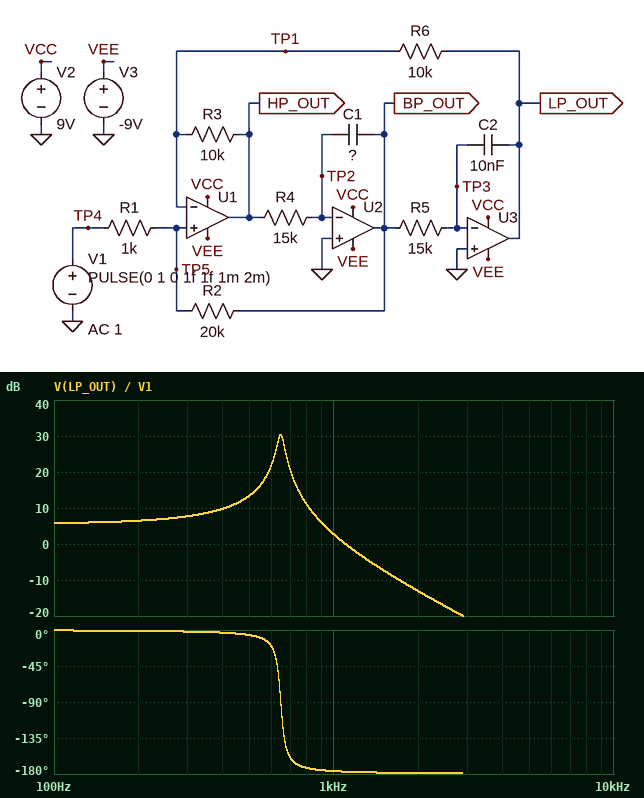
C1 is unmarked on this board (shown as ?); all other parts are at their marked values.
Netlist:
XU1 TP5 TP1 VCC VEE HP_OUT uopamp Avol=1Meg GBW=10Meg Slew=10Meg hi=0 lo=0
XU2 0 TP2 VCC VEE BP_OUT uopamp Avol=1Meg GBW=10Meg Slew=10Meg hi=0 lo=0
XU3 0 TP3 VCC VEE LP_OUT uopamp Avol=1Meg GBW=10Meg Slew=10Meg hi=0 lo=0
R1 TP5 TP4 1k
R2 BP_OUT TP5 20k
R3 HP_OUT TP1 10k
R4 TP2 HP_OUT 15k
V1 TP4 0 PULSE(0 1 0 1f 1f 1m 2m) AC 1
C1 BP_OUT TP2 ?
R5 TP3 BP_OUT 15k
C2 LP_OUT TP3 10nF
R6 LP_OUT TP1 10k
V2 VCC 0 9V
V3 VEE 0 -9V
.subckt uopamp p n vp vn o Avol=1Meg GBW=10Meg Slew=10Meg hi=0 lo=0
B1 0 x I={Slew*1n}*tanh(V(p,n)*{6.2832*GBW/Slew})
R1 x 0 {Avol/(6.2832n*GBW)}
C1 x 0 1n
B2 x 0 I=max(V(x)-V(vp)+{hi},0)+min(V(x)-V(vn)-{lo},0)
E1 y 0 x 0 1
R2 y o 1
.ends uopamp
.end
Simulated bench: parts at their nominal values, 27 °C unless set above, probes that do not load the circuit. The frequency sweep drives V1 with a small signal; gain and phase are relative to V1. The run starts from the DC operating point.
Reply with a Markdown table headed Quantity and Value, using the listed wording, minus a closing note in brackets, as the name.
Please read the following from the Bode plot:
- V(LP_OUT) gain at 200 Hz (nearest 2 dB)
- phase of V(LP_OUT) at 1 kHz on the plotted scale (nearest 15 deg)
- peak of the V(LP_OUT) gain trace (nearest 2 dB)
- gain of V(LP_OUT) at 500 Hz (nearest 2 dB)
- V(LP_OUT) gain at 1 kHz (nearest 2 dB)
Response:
| Quantity | Value |
|---|---|
| V(LP_OUT) gain at 200 Hz | 6 dB |
| phase of V(LP_OUT) at 1 kHz on the plotted scale | -180 deg |
| peak of the V(LP_OUT) gain trace | 30 dB |
| gain of V(LP_OUT) at 500 Hz | 14 dB |
| V(LP_OUT) gain at 1 kHz | 2 dB |
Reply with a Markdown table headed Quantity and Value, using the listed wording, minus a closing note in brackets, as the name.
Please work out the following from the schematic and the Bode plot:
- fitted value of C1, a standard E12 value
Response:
| Quantity | Value |
|---|---|
| fitted value of C1, a standard E12 value | 27 nF |
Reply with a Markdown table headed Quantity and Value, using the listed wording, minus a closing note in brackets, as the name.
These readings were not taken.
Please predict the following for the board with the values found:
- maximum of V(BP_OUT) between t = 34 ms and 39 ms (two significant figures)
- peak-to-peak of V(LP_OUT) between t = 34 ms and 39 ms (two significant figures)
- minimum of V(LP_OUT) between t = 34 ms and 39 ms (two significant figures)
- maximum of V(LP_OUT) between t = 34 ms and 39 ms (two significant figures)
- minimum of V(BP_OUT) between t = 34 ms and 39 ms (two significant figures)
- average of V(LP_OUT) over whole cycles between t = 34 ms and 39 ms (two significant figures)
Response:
| Quantity | Value |
|---|---|
| maximum of V(BP_OUT) between t = 34 ms and 39 ms | 1.4 V |
| peak-to-peak of V(LP_OUT) between t = 34 ms and 39 ms | 6.2 V |
| minimum of V(LP_OUT) between t = 34 ms and 39 ms | -2.2 V |
| maximum of V(LP_OUT) between t = 34 ms and 39 ms | 4.1 V |
| minimum of V(BP_OUT) between t = 34 ms and 39 ms | -1.4 V |
| average of V(LP_OUT) over whole cycles between t = 34 ms and 39 ms | 950 mV |
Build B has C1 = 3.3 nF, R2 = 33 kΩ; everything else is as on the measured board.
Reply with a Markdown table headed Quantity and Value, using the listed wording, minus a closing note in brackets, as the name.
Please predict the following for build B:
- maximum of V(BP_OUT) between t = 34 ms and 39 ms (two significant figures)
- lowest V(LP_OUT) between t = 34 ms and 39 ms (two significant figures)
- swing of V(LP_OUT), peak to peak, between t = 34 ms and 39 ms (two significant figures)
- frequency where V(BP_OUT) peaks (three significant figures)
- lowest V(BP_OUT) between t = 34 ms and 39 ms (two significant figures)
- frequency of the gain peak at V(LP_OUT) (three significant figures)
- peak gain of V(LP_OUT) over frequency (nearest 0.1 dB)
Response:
| Quantity | Value |
|---|---|
| maximum of V(BP_OUT) between t = 34 ms and 39 ms | 2.3 V |
| lowest V(LP_OUT) between t = 34 ms and 39 ms | -1.2 V |
| swing of V(LP_OUT), peak to peak, between t = 34 ms and 39 ms | 4.4 V |
| frequency where V(BP_OUT) peaks | 1.85 kHz |
| lowest V(BP_OUT) between t = 34 ms and 39 ms | -2.3 V |
| frequency of the gain peak at V(LP_OUT) | 1.84 kHz |
| peak gain of V(LP_OUT) over frequency | 25.6 dB |
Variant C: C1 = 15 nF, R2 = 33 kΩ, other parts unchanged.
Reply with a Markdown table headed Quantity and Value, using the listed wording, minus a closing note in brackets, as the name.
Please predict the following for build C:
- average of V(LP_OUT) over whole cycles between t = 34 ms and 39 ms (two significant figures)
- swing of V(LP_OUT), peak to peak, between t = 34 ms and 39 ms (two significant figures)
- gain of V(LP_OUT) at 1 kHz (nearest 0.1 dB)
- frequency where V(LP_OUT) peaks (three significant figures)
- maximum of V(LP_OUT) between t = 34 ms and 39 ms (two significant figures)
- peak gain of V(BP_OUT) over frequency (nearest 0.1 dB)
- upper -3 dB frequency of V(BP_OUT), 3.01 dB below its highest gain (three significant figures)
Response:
| Quantity | Value |
|---|---|
| average of V(LP_OUT) over whole cycles between t = 34 ms and 39 ms | 970 mV |
| swing of V(LP_OUT), peak to peak, between t = 34 ms and 39 ms | 4.1 V |
| gain of V(LP_OUT) at 1 kHz | 15.2 dB |
| frequency where V(LP_OUT) peaks | 866 Hz |
| maximum of V(LP_OUT) between t = 34 ms and 39 ms | 3.0 V |
| peak gain of V(BP_OUT) over frequency | 30.4 dB |
| upper -3 dB frequency of V(BP_OUT), 3.01 dB below its highest gain | 887 Hz |
